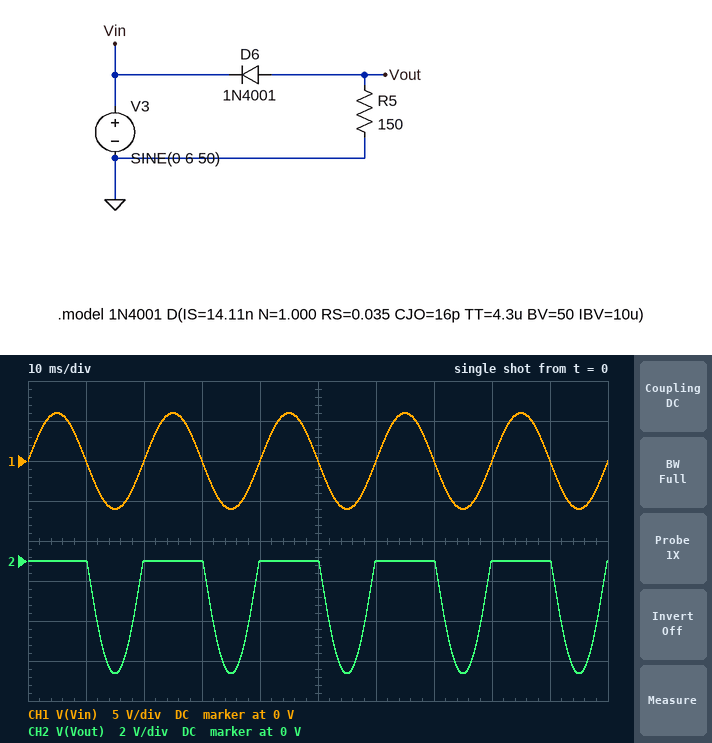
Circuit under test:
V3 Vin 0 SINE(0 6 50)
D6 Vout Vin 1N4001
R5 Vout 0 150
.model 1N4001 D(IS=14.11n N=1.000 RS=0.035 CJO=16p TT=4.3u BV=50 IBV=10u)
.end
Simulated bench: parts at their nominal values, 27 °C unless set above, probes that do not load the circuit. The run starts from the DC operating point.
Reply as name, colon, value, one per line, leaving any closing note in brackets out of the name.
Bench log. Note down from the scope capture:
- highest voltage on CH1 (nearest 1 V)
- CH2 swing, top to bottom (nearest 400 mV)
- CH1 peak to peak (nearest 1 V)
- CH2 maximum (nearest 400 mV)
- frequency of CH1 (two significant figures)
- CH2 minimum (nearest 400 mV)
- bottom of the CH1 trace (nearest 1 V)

highest voltage on CH1: 6 V
CH2 swing, top to bottom: 5.6 V
CH1 peak to peak: 12 V
CH2 maximum: 0 V
frequency of CH1: 50 Hz
CH2 minimum: -5.6 V
bottom of the CH1 trace: -6 V
